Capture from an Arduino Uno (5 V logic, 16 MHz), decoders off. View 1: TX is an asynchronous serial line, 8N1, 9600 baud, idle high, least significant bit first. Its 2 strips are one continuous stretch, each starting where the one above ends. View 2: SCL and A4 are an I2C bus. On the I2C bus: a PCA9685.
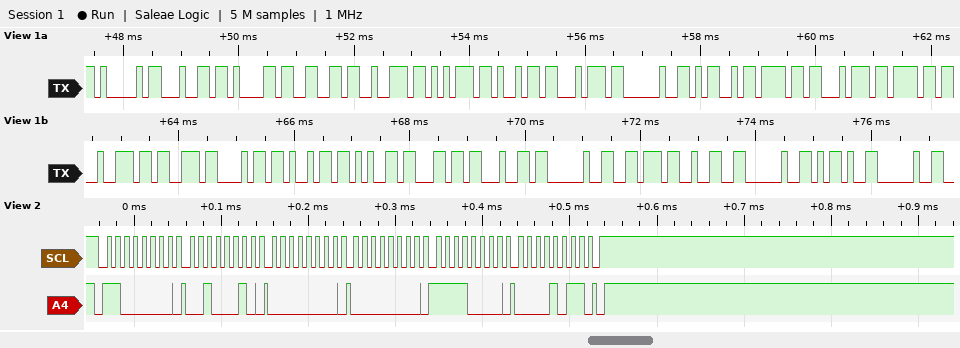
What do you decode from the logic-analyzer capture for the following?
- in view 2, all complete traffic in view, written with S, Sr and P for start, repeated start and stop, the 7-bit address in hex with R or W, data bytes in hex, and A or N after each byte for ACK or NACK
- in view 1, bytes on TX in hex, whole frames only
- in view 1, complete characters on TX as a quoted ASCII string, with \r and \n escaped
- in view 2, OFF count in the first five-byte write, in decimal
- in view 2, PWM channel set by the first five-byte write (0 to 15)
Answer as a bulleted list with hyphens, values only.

- S 60W A 22 A 00 A 00 A F0 A 0B A P
- 0x41 0x64 0x61 0x66 0x72 0x75 0x69 0x74 0x20 0x4D 0x6F 0x74 0x6F 0x72 0x73 0x68 0x69 0x65 0x6C 0x64 0x20 0x76 0x32 0x20 0x2D 0x20
- "Adafruit Motorshield v2 - "
- 3056
- 7
